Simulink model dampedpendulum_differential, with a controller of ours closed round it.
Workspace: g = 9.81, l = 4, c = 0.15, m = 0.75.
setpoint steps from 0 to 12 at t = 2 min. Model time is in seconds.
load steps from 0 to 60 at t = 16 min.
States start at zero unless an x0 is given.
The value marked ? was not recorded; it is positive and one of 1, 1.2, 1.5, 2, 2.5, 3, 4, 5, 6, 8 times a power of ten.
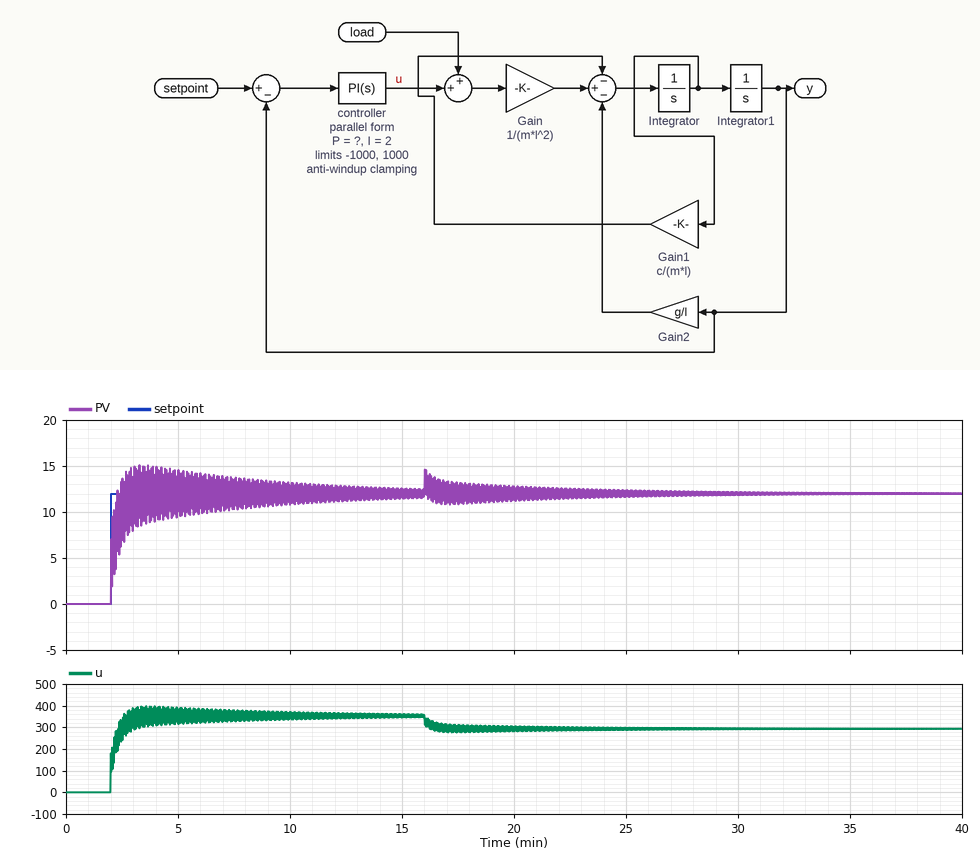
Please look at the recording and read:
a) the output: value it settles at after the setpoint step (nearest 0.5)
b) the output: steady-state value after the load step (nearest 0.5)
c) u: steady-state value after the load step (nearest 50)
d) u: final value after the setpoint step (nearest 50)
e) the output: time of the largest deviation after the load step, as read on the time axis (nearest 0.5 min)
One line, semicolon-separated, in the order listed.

12.0; 12.0; 300; 350; 16.0 min
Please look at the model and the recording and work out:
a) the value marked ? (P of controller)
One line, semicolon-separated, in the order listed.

15
